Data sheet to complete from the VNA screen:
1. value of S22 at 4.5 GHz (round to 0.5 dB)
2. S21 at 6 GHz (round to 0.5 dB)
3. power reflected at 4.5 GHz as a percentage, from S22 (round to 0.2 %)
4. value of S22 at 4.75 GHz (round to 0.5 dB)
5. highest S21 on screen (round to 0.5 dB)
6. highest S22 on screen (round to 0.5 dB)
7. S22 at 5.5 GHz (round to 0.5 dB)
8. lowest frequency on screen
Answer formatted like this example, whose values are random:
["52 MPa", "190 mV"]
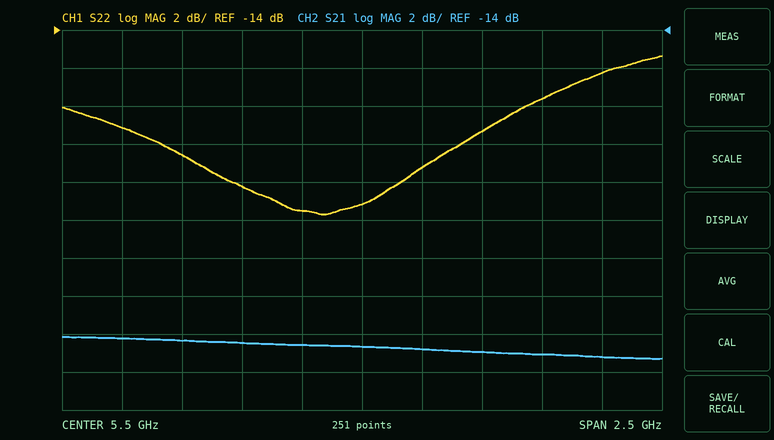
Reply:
["-19.0 dB", "-31.0 dB", "1.2 %", "-20.5 dB", "-30.0 dB", "-15.5 dB", "-23.0 dB", "4.25 GHz"]
